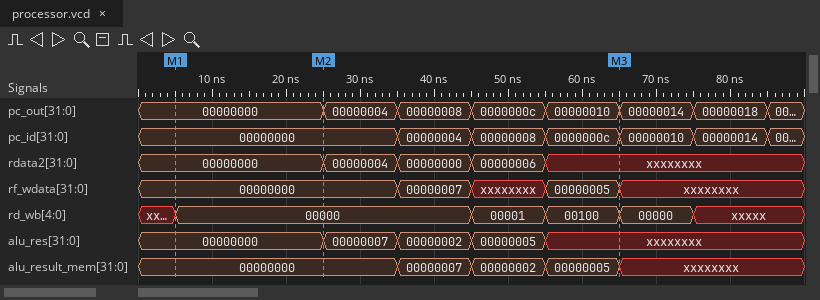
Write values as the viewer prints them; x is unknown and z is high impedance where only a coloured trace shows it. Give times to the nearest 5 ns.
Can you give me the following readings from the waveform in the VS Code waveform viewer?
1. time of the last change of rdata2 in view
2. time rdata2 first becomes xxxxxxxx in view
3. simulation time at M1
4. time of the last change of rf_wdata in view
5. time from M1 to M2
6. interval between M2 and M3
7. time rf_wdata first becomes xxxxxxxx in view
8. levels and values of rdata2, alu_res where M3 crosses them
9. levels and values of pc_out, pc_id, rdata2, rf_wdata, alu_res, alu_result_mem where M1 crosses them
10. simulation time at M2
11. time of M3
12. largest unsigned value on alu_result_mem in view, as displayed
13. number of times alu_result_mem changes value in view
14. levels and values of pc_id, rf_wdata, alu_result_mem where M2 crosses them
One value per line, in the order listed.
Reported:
55 ns
55 ns
5 ns
65 ns
20 ns
40 ns
45 ns
rdata2=xxxxxxxx, alu_res=xxxxxxxx
pc_out=00000000, pc_id=00000000, rdata2=00000000, rf_wdata=00000000, alu_res=00000000, alu_result_mem=00000000
25 ns
65 ns
00000007
4
pc_id=00000000, rf_wdata=00000000, alu_result_mem=00000000
